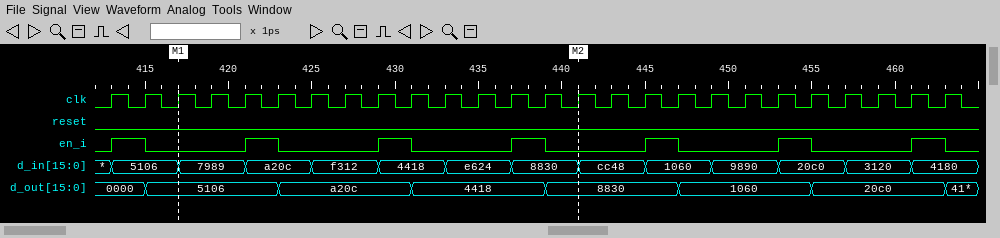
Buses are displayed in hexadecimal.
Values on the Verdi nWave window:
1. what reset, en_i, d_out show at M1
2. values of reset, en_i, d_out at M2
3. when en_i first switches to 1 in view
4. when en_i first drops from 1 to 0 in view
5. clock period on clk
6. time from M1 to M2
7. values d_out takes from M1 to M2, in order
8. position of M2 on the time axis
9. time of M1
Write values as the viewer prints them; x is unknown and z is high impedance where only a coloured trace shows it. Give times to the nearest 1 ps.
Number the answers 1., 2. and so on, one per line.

1. reset=0, en_i=0, d_out=5106
2. reset=0, en_i=0, d_out=8830
3. 413 ps
4. 415 ps
5. 2 ps
6. 24 ps
7. 5106, a20c, 4418, 8830
8. 441 ps
9. 417 ps
